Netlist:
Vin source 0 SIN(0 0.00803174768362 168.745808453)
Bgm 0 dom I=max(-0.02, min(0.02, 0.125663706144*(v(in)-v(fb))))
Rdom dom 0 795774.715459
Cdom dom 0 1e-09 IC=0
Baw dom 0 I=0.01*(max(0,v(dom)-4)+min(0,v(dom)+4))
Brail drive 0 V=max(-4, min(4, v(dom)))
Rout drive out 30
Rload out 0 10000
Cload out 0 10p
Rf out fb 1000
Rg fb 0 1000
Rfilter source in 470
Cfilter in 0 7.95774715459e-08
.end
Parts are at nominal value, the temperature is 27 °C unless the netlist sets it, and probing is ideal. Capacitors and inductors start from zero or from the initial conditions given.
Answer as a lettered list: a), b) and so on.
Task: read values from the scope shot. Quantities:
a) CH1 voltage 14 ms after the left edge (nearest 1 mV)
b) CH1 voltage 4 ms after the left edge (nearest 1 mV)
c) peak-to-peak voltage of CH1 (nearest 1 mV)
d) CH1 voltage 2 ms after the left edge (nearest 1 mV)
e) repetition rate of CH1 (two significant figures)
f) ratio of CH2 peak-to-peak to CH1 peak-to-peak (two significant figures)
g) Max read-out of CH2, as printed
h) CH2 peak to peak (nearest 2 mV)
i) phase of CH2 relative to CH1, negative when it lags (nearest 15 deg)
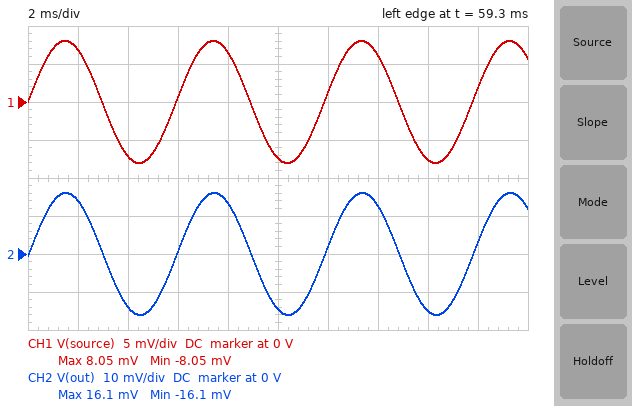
a) 6 mV
b) -7 mV
c) 16 mV
d) 7 mV
e) 170 Hz
f) 2.0
g) 16.1 mV
h) 32 mV
i) 0 deg
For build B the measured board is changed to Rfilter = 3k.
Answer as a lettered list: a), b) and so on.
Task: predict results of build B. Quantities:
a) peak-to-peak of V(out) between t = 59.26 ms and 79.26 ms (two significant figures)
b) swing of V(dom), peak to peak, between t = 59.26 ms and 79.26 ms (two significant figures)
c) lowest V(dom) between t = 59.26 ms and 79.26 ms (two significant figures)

a) 31 mV
b) 32 mV
c) -16 mV
